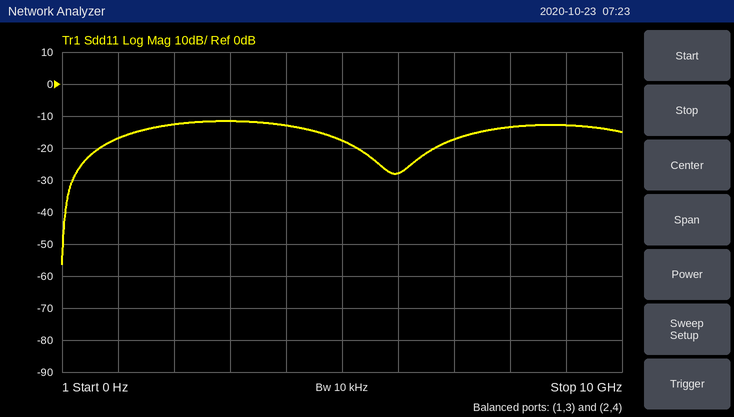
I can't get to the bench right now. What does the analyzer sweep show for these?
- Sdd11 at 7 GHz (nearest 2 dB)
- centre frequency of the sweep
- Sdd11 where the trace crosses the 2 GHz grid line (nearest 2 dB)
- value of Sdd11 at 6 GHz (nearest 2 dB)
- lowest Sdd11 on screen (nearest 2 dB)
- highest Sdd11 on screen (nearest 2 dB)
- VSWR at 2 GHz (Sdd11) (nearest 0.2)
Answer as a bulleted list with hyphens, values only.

- -18 dB
- 5 GHz
- -12 dB
- -28 dB
- -56 dB
- -12 dB
- 1.6
